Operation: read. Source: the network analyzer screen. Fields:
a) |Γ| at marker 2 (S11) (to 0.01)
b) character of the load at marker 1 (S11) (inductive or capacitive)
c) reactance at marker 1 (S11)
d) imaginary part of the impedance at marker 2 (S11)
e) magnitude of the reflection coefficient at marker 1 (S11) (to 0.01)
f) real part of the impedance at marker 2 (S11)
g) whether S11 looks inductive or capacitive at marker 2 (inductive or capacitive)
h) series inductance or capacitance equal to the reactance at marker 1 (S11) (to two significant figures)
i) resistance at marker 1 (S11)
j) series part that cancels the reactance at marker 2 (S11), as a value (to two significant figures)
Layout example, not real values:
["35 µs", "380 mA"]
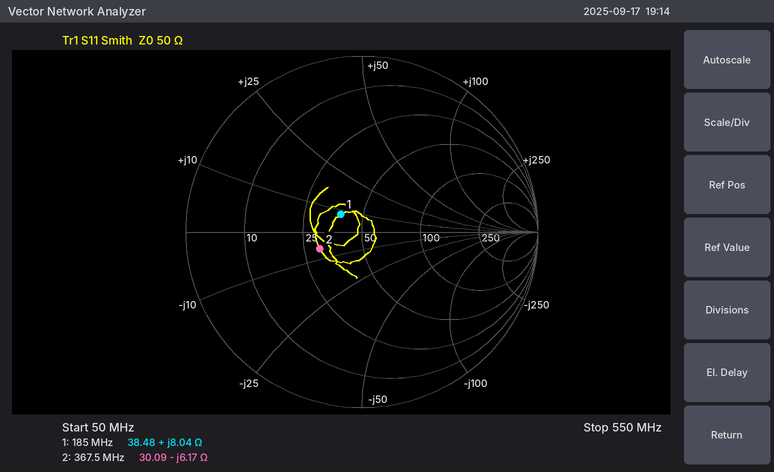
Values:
["0.26", "inductive", "+8.04 Ω", "-6.17 Ω", "0.16", "30.09 Ω", "capacitive", "6.9 nH", "38.48 Ω", "2.7 nH"]
